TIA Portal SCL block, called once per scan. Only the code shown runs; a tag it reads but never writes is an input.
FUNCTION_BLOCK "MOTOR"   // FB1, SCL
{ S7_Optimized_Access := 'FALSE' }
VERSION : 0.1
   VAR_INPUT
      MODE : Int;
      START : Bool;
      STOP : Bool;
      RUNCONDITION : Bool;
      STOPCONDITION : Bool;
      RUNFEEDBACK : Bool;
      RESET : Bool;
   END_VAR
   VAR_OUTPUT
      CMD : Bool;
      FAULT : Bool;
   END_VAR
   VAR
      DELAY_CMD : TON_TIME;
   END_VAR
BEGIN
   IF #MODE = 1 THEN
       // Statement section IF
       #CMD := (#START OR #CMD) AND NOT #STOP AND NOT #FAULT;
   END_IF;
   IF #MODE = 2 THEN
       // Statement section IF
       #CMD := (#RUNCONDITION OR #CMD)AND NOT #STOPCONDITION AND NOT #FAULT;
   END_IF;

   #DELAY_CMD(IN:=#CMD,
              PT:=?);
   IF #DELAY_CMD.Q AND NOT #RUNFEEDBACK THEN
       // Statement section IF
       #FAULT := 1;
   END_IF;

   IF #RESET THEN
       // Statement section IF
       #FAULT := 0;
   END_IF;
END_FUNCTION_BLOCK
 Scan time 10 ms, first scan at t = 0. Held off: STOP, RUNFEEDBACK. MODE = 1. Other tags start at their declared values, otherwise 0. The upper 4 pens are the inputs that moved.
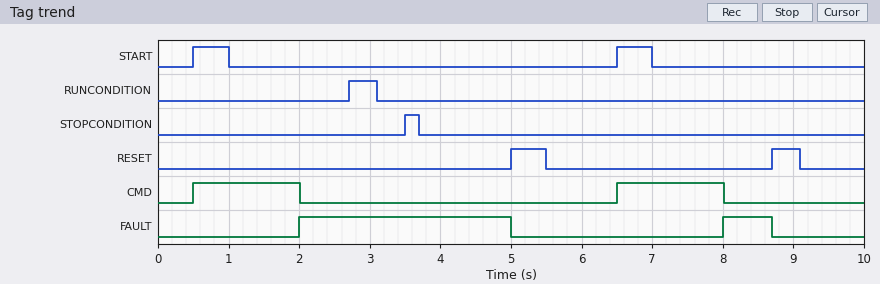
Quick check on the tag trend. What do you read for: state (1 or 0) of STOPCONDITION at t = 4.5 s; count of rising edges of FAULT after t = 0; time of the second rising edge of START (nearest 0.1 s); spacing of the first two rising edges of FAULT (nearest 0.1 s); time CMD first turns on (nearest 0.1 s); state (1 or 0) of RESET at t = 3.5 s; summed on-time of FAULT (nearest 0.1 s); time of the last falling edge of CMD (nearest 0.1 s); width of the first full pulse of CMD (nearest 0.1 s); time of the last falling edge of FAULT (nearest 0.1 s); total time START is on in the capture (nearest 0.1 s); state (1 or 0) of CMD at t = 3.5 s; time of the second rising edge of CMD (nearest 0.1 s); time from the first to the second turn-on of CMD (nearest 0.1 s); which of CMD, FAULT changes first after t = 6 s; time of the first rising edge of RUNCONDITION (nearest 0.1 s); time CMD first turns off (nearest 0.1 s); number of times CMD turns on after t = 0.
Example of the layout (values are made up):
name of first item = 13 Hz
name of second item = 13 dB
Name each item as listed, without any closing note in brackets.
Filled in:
state (1 or 0) of STOPCONDITION at t = 4.5 s = 0
count of rising edges of FAULT after t = 0 = 2
time of the second rising edge of START = 6.5 s
spacing of the first two rising edges of FAULT = 6.0 s
time CMD first turns on = 0.5 s
state (1 or 0) of RESET at t = 3.5 s = 0
summed on-time of FAULT = 3.7 s
time of the last falling edge of CMD = 8.0 s
width of the first full pulse of CMD = 1.5 s
time of the last falling edge of FAULT = 8.7 s
total time START is on in the capture = 1.0 s
state (1 or 0) of CMD at t = 3.5 s = 0
time of the second rising edge of CMD = 6.5 s
time from the first to the second turn-on of CMD = 6.0 s
which of CMD, FAULT changes first after t = 6 s = CMD
time of the first rising edge of RUNCONDITION = 2.7 s
time CMD first turns off = 2.0 s
number of times CMD turns on after t = 0 = 2
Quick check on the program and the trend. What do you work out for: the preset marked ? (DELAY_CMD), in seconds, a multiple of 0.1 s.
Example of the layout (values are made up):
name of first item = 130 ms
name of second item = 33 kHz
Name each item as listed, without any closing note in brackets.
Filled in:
the preset marked ? (DELAY_CMD), in seconds, a multiple of 0.1 s = 1.5 s
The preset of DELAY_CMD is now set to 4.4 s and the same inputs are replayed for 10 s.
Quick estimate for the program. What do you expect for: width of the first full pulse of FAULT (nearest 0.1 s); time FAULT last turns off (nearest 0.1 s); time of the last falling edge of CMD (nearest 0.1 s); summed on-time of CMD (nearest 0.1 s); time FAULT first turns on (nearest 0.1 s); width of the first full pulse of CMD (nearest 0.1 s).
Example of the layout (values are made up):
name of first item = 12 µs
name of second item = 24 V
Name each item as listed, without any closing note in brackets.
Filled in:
width of the first full pulse of FAULT = 0.1 s
time FAULT last turns off = 5.0 s
time of the last falling edge of CMD = 4.9 s
summed on-time of CMD = 7.9 s
time FAULT first turns on = 4.9 s
width of the first full pulse of CMD = 4.4 s
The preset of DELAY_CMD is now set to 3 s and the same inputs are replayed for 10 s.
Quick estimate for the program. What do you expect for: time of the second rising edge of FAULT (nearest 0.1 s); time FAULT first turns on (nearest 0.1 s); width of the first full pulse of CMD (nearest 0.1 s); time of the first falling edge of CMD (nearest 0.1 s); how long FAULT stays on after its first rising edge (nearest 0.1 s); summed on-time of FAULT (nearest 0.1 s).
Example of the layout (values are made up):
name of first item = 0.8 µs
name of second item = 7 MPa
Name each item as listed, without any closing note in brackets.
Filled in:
time of the second rising edge of FAULT = 9.5 s
time FAULT first turns on = 3.5 s
width of the first full pulse of CMD = 3.0 s
time of the first falling edge of CMD = 3.5 s
how long FAULT stays on after its first rising edge = 1.5 s
summed on-time of FAULT = 2.0 s
